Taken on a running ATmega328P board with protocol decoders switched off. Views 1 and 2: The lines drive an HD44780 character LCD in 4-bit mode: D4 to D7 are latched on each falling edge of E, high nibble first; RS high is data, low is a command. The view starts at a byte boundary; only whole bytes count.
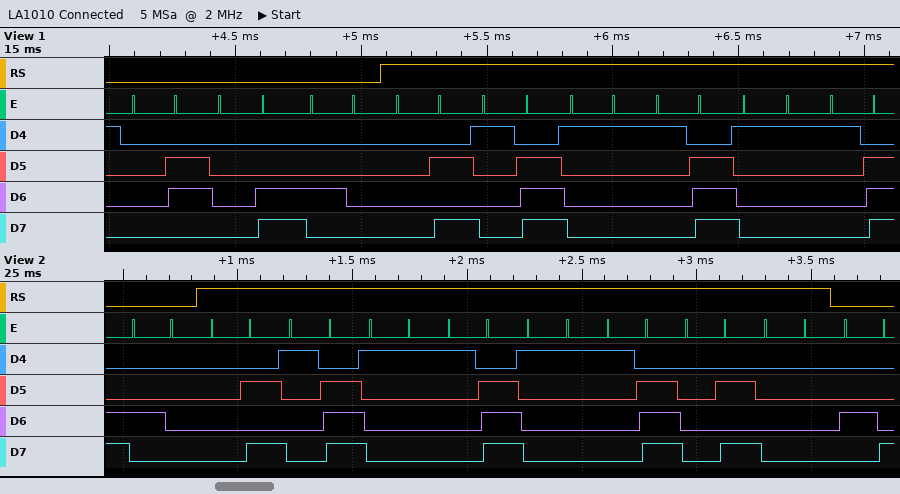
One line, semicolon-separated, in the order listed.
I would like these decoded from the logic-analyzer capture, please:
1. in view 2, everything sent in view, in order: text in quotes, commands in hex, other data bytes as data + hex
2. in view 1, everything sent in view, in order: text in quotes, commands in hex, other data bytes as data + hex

0x40 data 0A 1E 11 1E 11 1E 0A 00 0x48; 0x06 0x0C 0x40 data 0A 1E 11 1E 11 1E
